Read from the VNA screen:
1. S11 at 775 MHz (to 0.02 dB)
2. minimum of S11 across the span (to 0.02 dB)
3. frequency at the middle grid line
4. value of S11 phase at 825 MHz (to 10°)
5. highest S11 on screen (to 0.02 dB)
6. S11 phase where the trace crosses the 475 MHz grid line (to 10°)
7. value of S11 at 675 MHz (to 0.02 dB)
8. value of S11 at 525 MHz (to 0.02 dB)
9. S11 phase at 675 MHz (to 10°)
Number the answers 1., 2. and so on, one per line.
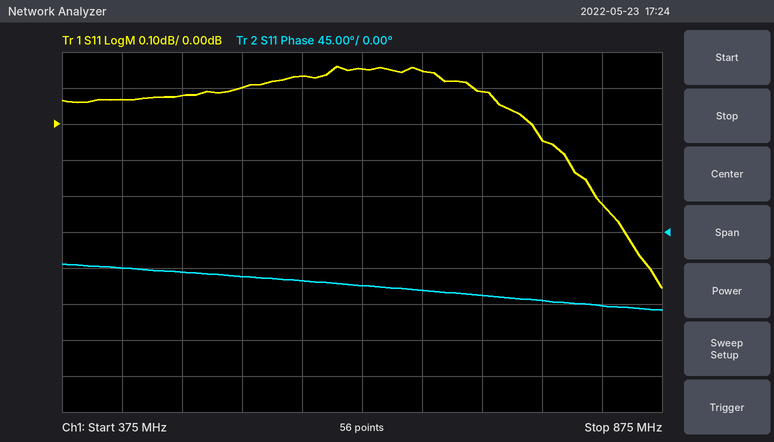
1. -0.04 dB
2. -0.46 dB
3. 625 MHz
4. -90°
5. 0.16 dB
6. -50°
7. 0.14 dB
8. 0.10 dB
9. -70°
